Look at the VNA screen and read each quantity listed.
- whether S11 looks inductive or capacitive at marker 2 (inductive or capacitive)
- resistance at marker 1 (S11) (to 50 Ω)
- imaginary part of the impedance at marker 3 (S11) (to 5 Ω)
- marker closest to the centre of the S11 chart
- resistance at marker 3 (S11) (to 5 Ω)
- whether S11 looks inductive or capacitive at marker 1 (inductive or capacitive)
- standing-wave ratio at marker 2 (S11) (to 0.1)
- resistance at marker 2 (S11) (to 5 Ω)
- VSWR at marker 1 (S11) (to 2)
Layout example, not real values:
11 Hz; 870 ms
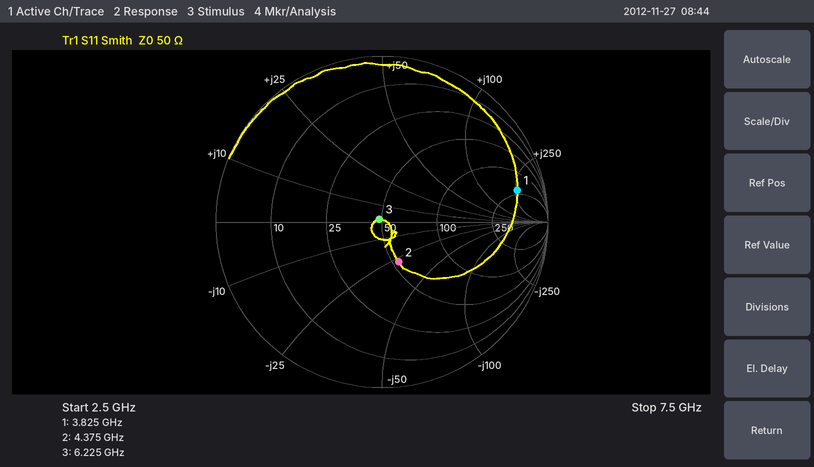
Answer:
capacitive; 200 Ω; 0 Ω; marker 3; 50 Ω; inductive; 1.7; 55 Ω; 12
